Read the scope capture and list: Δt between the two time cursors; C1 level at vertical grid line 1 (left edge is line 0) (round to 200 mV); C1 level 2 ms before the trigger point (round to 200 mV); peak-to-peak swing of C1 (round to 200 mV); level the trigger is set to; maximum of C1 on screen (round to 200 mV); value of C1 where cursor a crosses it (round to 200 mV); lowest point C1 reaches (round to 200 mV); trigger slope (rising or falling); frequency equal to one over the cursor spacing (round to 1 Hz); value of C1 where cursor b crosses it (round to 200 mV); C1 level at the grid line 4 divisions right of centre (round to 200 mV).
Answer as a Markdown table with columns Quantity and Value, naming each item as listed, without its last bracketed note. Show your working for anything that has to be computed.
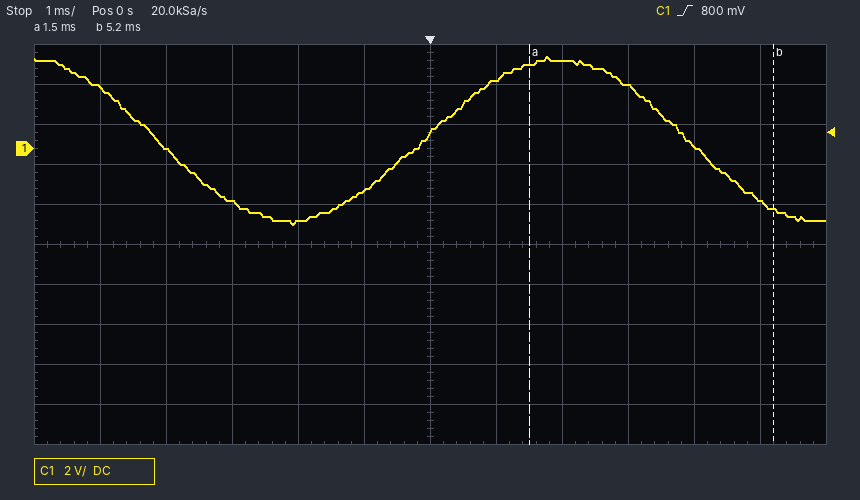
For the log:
| Quantity | Value |
|---|---|
| Δt between the two time cursors | 5.2 ms − (1.5 ms) = 3.7 ms |
| C1 level at vertical grid line 1 (left edge is line 0) | 3.0 V |
| C1 level 2 ms before the trigger point | -3.6 V |
| peak-to-peak swing of C1 | 4.6 V − (-3.8 V) = 8.4 V |
| level the trigger is set to | 800 mV |
| maximum of C1 on screen | 4.6 V |
| value of C1 where cursor a crosses it | 4.2 V |
| lowest point C1 reaches | -3.8 V |
| trigger slope | rising |
| frequency equal to one over the cursor spacing | 1 / 3.7 ms ≈ 270 Hz |
| value of C1 where cursor b crosses it | -3.0 V |
| C1 level at the grid line 4 divisions right of centre | 200 mV |
